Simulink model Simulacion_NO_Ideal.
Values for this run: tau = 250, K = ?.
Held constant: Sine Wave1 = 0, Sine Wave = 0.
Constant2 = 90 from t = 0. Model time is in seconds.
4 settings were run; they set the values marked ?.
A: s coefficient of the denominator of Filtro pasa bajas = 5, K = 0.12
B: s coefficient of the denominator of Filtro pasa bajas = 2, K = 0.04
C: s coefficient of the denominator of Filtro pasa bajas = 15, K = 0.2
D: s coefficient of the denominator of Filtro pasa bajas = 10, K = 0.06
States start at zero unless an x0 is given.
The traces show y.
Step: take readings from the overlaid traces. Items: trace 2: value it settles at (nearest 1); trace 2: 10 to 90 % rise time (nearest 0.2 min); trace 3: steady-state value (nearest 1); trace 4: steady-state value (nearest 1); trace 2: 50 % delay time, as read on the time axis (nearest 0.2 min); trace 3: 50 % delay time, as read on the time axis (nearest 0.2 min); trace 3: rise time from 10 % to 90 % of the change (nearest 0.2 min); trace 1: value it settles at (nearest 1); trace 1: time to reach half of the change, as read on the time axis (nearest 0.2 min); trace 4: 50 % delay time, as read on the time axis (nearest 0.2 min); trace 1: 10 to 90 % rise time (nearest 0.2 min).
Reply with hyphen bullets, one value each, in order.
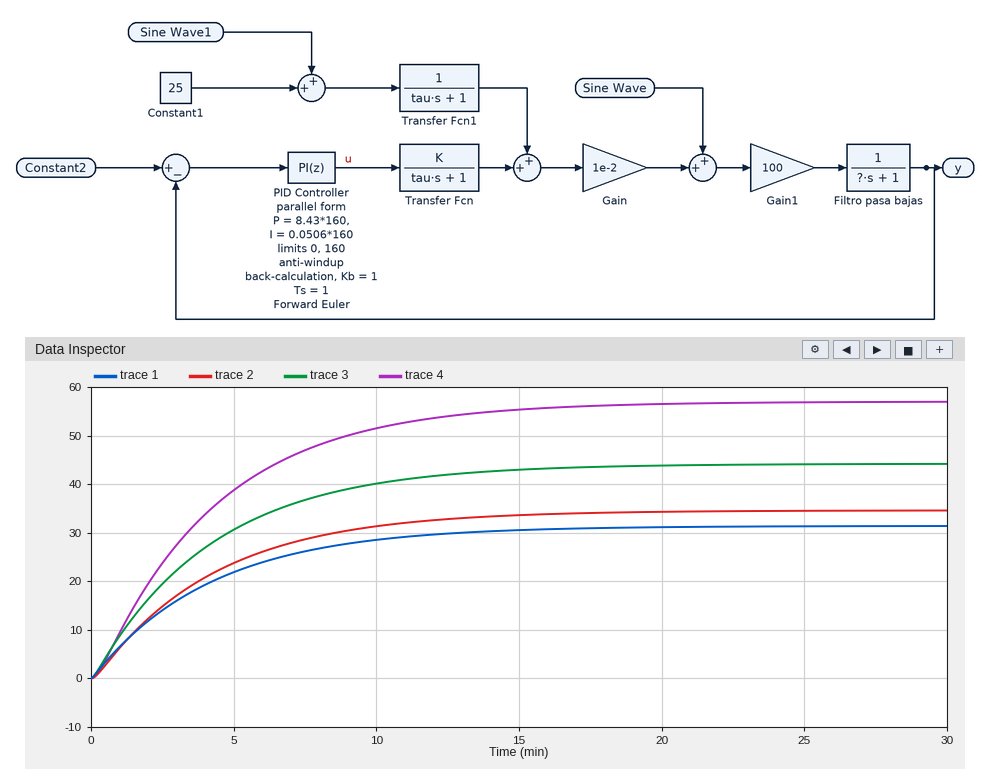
- 35
- 9.2 min
- 44
- 57
- 3.0 min
- 3.0 min
- 9.2 min
- 31
- 3.0 min
- 3.2 min
- 9.2 min
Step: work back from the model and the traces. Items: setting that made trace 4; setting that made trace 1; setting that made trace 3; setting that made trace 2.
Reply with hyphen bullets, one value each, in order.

- C
- B
- A
- D
